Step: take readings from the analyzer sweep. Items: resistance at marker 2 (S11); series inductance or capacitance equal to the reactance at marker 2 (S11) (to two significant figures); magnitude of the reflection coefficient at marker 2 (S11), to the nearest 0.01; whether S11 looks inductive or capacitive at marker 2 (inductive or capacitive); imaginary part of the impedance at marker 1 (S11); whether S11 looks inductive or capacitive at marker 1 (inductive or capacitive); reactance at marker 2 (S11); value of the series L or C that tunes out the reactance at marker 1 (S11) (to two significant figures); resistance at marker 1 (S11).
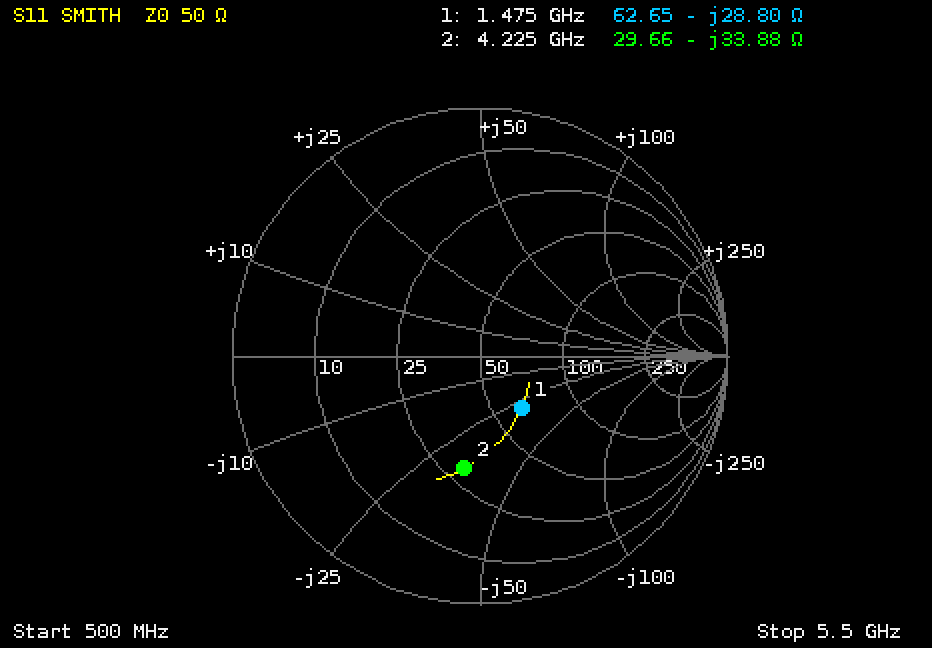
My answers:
29.66 Ω
1.1 pF
0.46
capacitive
-28.80 Ω
capacitive
-33.88 Ω
3.1 nH
62.65 Ω
